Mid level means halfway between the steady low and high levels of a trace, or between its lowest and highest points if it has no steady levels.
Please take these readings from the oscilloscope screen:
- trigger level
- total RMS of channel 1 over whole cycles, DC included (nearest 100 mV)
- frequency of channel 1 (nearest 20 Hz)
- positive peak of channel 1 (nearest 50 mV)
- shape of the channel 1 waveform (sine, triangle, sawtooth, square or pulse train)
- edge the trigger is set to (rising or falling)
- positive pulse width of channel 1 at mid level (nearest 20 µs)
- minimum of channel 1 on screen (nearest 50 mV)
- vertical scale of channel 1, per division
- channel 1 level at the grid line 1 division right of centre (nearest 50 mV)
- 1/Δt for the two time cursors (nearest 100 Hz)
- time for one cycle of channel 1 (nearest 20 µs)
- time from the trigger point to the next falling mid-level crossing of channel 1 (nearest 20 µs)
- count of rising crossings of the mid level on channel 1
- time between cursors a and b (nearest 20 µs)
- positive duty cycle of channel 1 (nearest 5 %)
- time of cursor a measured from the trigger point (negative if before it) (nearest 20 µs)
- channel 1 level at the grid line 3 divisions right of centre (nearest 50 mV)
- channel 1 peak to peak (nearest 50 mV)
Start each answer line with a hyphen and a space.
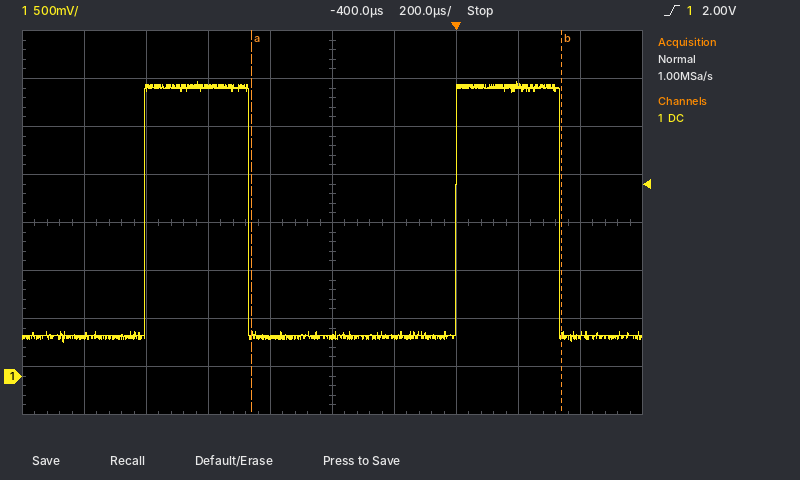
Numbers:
- 2.00 V
- 1.8 V
- 1.00 kHz
- 3.05 V
- pulse train
- rising
- 340 µs
- 350 mV
- 500 mV
- 400 mV
- 1.0 kHz
- 1.00 ms
- 340 µs
- 2
- 1.00 ms
- 35 %
- -660 µs
- 3.05 V
- 2.70 V
